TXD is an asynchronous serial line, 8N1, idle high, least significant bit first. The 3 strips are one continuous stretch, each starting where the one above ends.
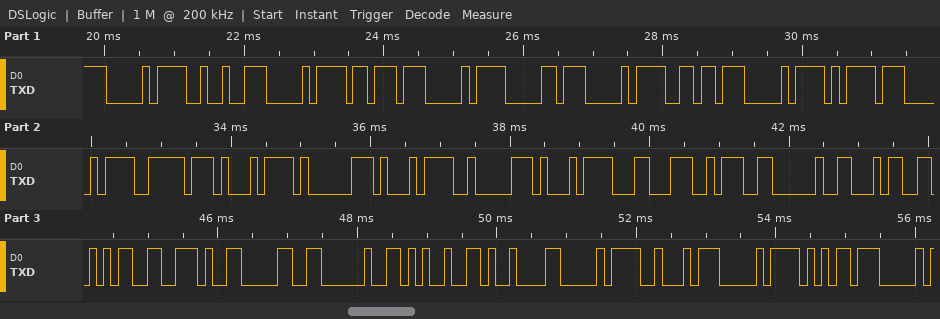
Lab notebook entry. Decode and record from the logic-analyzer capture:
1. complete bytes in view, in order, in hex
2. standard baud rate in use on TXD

D0 92 D0 BB D0 B0 D0 B6 D0 BD D0 BE D1 81 D1 82 D1 8C 3A 20 34 35 2E 30 20 25 09 D0 A2 D0 B5
9600 baud
